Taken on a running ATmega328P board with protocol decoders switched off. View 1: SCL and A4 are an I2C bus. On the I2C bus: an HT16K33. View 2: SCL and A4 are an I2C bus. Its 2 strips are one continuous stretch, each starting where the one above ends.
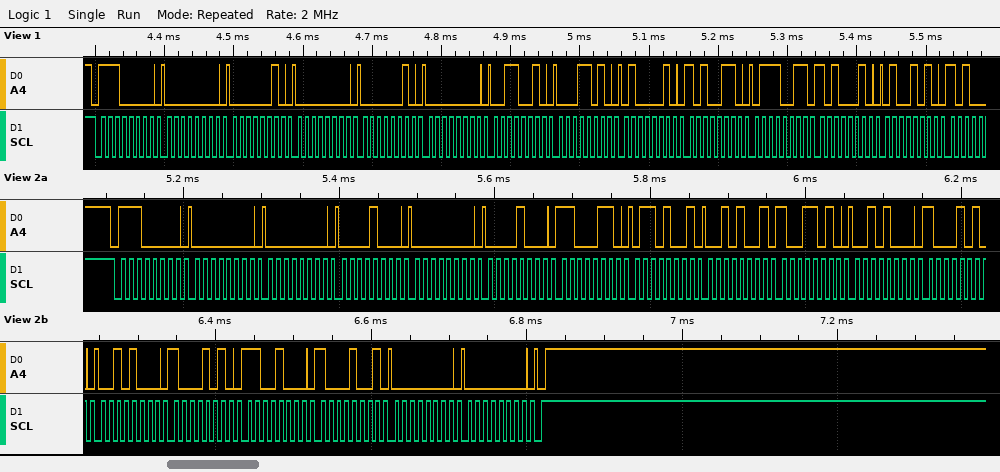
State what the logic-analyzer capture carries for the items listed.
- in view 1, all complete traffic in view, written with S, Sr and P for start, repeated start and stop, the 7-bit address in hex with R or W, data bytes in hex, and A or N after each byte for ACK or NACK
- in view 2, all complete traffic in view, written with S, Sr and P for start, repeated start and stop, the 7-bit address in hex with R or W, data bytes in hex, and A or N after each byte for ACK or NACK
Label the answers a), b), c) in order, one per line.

a) S 70W A 00 A 02 A 00 A 02 A 00 A 32 A 1A A 42 A A6 A 73 A A2 A 4A A
b) S 70W A 00 A 00 A 08 A 00 A 08 A C6 A 69 A 29 A 9A A 28 A 8A A 28 A 8A A C8 A 89 A 00 A 00 A P
